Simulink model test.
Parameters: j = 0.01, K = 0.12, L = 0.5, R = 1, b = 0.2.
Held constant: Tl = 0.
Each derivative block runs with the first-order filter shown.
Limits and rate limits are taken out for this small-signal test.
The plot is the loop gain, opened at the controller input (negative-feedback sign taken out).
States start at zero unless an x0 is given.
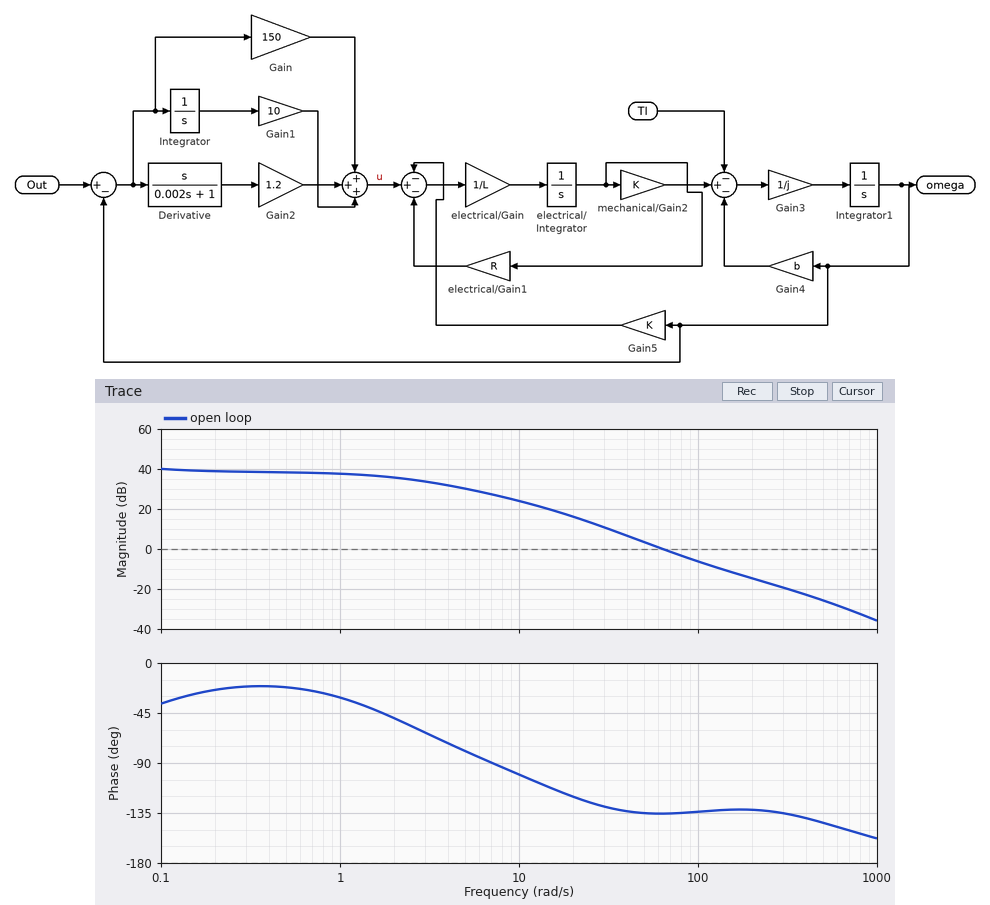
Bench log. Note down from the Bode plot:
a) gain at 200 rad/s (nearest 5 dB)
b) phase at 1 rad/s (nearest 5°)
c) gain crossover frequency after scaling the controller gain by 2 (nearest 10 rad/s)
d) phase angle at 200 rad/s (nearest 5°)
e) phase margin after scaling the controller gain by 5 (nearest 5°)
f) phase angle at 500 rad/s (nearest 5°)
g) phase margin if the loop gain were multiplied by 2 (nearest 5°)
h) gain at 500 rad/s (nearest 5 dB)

-15 dB
-30°
100 rad/s
-130°
50°
-145°
45°
-25 dB
